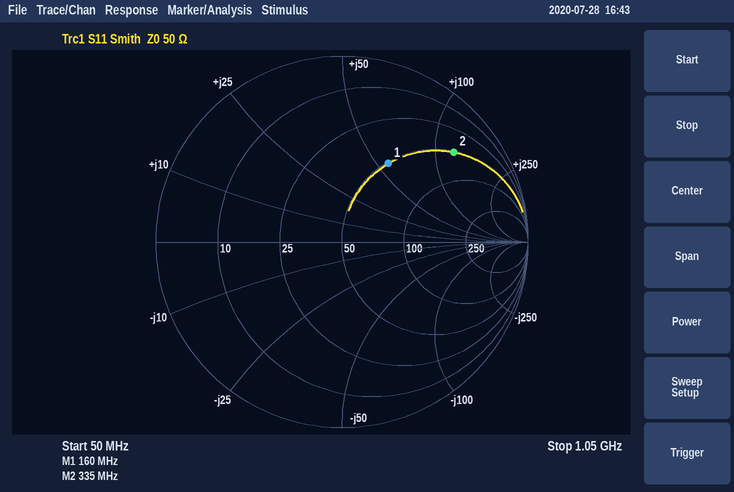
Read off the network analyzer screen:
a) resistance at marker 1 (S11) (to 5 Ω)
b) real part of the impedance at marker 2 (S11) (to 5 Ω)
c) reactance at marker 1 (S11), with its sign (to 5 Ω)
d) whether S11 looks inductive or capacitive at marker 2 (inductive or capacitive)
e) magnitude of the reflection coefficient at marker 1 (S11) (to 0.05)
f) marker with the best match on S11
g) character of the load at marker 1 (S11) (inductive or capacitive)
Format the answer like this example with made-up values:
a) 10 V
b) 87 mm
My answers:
a) 50 Ω
b) 50 Ω
c) +55 Ω
d) inductive
e) 0.50
f) marker 1
g) inductive
